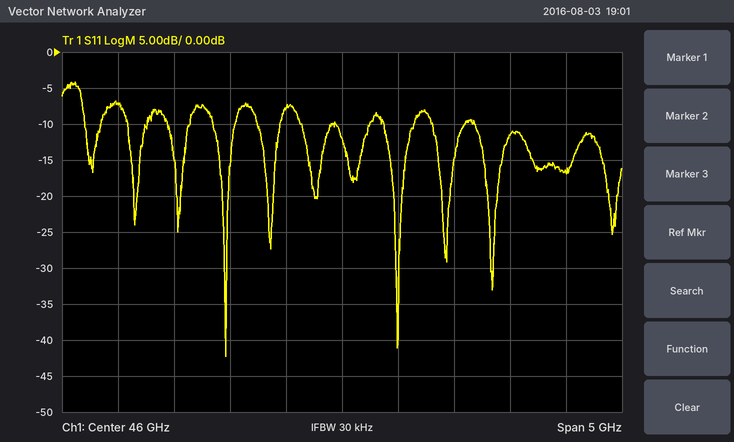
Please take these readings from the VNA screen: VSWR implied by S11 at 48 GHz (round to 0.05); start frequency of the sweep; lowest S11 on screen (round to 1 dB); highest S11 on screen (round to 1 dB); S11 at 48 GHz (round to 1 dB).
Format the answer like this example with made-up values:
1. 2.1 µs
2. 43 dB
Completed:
1. 1.35
2. 43.5 GHz
3. -42 dB
4. -4 dB
5. -17 dB
